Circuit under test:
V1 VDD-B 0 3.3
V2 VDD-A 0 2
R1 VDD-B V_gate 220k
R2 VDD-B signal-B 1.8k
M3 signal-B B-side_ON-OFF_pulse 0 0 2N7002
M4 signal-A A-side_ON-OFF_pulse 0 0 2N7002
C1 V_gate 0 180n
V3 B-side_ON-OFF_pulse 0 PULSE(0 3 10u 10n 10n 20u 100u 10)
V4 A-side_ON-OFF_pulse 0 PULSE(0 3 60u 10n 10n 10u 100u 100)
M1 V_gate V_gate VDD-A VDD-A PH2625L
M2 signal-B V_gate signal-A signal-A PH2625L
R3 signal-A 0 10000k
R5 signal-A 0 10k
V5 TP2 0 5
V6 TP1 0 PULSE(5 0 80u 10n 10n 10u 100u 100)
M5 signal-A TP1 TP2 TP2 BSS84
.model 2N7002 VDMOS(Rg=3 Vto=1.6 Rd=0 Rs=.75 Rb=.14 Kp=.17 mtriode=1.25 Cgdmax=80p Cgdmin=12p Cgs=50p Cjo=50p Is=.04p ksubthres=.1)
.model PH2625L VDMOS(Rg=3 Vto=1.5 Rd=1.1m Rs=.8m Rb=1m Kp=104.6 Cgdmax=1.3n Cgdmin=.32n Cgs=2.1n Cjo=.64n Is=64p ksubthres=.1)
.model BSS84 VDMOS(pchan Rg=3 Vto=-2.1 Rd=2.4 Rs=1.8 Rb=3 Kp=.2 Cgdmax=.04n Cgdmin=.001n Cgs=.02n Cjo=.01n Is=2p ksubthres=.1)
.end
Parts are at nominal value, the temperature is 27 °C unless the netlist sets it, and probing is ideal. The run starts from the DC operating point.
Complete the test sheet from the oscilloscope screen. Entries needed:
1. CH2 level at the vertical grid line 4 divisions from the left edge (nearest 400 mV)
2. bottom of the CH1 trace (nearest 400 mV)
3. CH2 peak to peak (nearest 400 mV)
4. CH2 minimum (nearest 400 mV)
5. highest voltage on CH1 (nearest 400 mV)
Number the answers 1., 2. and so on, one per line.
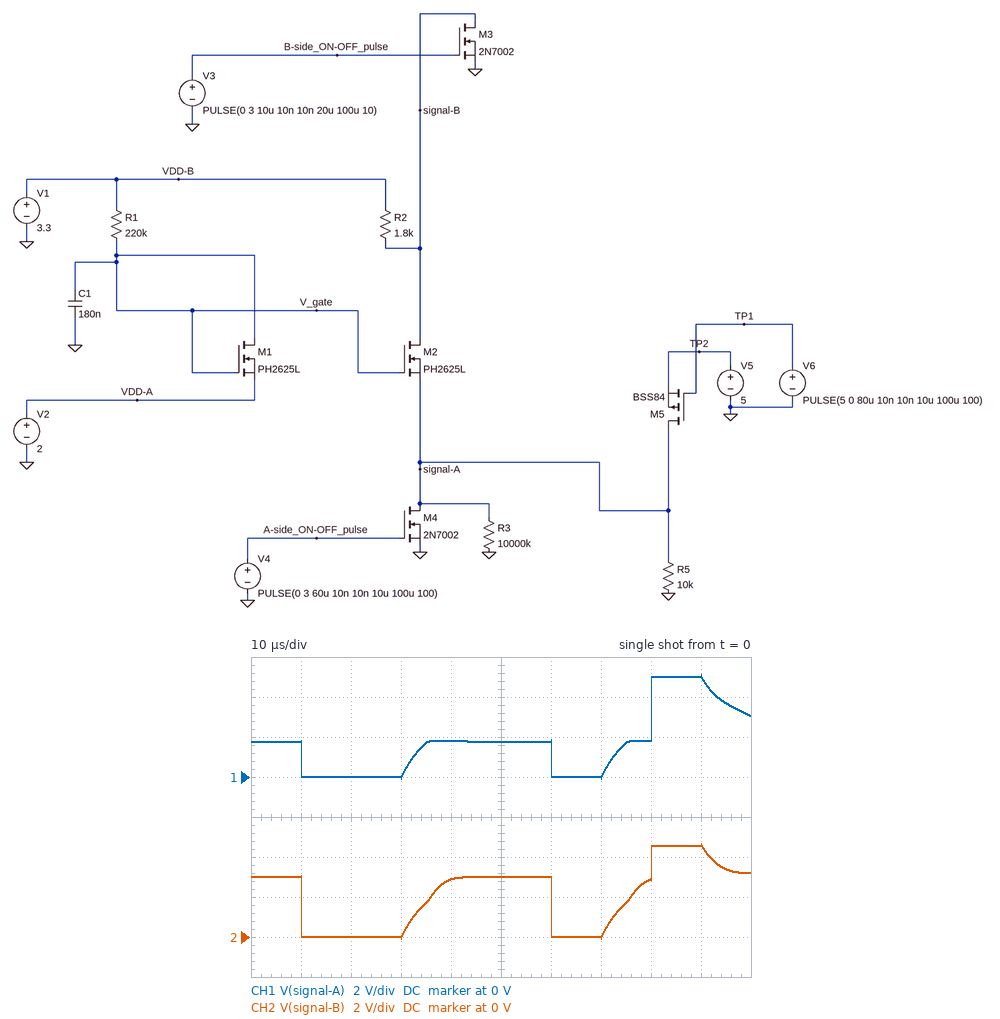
1. 2.8 V
2. 0 V
3. 4.8 V
4. 0 V
5. 5.2 V
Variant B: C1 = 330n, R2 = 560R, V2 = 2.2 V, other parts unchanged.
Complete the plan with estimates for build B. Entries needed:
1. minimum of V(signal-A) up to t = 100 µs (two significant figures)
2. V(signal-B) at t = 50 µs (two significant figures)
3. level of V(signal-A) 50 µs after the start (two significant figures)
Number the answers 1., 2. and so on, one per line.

1. -54 mV
2. 3.2 V
3. 1.9 V
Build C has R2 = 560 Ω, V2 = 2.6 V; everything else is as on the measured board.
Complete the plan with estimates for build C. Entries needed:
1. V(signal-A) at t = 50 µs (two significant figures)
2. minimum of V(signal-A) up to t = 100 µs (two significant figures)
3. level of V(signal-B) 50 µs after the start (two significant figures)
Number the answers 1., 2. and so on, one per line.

1. 2.2 V
2. -54 mV
3. 3.2 V
